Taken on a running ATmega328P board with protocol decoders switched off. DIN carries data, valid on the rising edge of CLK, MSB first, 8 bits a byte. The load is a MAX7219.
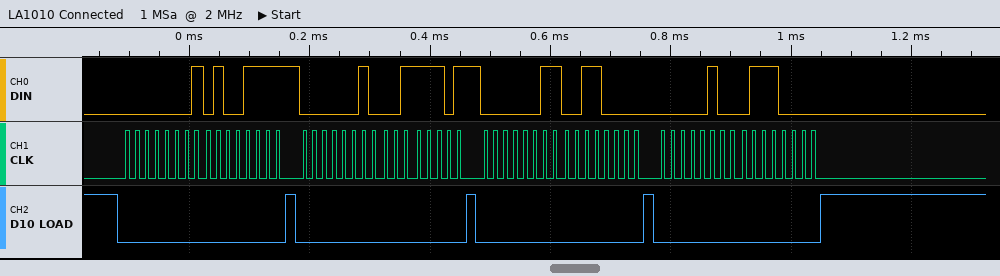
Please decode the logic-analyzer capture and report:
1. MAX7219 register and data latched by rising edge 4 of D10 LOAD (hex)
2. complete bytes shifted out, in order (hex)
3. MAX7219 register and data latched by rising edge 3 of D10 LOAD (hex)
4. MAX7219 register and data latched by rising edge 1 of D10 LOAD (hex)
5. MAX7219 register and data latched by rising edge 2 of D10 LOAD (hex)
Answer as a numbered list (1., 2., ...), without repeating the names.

1. register 0x4, data 0x70
2. 0x01 0x4F 0x02 0x3D 0x03 0x30 0x04 0x70
3. register 0x3, data 0x30
4. register 0x1, data 0x4F
5. register 0x2, data 0x3D
